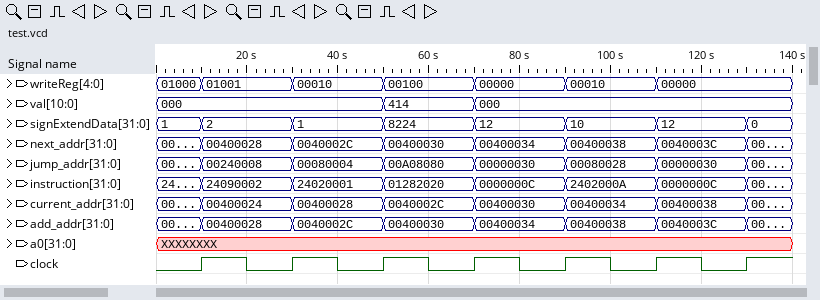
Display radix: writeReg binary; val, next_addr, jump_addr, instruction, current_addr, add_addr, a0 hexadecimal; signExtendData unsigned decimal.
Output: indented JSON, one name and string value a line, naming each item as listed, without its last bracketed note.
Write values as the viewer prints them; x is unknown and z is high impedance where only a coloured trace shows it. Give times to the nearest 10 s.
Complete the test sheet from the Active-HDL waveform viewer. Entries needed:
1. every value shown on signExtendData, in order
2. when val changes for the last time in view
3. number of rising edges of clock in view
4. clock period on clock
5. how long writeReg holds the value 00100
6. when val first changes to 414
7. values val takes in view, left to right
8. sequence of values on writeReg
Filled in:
{
  "every value shown on signExtendData, in order": "1, 2, 1, 8224, 12, 10, 12, 0",
  "when val changes for the last time in view": "70 s",
  "number of rising edges of clock in view": "7",
  "clock period on clock": "20 s",
  "how long writeReg holds the value 00100": "20 s",
  "when val first changes to 414": "50 s",
  "values val takes in view, left to right": "000, 414, 000",
  "sequence of values on writeReg": "01000, 01001, 00010, 00100, 00000, 00010, 00000"
}
